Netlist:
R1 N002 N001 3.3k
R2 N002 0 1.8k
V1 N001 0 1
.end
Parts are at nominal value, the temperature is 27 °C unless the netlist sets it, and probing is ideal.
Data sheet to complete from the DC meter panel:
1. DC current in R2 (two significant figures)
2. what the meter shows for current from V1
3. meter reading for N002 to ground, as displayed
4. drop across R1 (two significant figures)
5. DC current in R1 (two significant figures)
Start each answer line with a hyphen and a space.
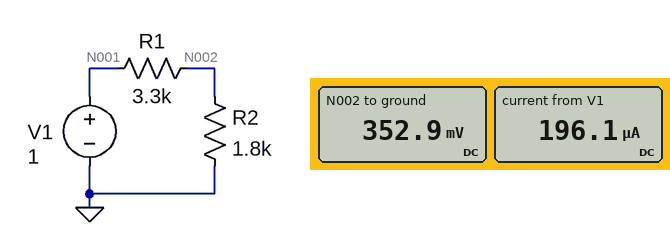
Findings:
- 200 µA
- 196.1 µA
- 352.9 mV
- 650 mV
- 200 µA
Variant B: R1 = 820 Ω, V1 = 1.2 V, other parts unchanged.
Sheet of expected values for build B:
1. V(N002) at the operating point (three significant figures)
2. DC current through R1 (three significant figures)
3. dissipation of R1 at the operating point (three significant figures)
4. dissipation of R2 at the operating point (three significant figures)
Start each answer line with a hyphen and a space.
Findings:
- 824 mV
- 458 µA
- 172 µW
- 378 µW
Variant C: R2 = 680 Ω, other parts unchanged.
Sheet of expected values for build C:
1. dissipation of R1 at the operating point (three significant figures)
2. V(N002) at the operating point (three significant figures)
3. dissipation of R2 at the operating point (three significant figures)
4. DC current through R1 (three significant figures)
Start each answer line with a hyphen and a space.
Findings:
- 208 µW
- 171 mV
- 42.9 µW
- 251 µA
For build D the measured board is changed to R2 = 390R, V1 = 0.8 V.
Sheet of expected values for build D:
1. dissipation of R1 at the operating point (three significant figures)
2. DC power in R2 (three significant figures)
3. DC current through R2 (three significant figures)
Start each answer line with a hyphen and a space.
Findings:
- 155 µW
- 18.3 µW
- 217 µA
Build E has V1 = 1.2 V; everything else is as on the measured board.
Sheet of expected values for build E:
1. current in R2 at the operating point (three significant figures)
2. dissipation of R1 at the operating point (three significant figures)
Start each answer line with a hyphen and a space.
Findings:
- 235 µA
- 183 µW
